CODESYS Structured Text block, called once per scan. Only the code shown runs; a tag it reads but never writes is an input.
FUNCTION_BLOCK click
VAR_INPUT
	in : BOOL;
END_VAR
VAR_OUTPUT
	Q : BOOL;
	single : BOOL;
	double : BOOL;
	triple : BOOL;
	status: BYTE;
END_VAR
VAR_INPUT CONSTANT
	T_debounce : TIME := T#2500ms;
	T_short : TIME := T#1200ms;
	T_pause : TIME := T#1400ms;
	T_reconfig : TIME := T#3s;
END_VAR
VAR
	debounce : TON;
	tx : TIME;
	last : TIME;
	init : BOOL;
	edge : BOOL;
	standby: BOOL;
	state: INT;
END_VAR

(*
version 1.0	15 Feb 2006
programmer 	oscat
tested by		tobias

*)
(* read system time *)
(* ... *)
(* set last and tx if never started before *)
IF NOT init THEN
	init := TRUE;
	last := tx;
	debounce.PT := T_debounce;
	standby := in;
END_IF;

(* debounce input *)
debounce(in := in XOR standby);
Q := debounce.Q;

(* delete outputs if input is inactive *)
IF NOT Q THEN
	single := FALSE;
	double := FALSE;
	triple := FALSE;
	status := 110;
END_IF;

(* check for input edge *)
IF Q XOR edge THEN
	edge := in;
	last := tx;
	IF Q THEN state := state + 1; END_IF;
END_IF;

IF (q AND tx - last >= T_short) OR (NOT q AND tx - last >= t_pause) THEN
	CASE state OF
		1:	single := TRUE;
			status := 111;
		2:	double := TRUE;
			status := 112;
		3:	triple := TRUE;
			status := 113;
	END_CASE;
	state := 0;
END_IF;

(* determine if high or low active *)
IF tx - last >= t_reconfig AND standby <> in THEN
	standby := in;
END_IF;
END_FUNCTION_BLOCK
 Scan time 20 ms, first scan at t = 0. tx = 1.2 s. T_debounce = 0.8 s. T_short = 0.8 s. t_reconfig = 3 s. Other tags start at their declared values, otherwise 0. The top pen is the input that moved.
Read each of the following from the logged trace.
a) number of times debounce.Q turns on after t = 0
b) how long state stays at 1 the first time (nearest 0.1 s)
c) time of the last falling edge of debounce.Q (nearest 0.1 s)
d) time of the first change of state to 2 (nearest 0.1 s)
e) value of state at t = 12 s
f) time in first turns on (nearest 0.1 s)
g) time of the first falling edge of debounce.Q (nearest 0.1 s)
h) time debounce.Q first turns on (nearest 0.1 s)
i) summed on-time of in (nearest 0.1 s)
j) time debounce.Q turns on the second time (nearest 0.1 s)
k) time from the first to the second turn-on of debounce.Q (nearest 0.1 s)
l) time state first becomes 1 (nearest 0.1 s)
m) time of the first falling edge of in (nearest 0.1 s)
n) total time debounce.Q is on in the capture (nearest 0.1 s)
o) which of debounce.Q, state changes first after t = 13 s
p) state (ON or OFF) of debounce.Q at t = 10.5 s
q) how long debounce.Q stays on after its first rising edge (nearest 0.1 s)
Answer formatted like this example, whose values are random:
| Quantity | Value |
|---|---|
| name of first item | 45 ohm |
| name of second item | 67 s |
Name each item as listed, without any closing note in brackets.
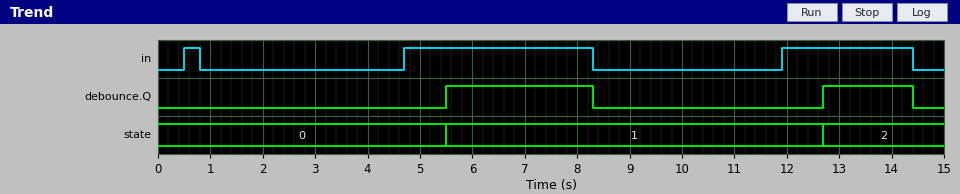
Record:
| Quantity | Value |
|---|---|
| number of times debounce.Q turns on after t = 0 | 2 |
| how long state stays at 1 the first time | 7.2 s |
| time of the last falling edge of debounce.Q | 14.4 s |
| time of the first change of state to 2 | 12.7 s |
| value of state at t = 12 s | 1 |
| time in first turns on | 0.5 s |
| time of the first falling edge of debounce.Q | 8.3 s |
| time debounce.Q first turns on | 5.5 s |
| summed on-time of in | 6.4 s |
| time debounce.Q turns on the second time | 12.7 s |
| time from the first to the second turn-on of debounce.Q | 7.2 s |
| time state first becomes 1 | 5.5 s |
| time of the first falling edge of in | 0.8 s |
| total time debounce.Q is on in the capture | 4.5 s |
| which of debounce.Q, state changes first after t = 13 s | debounce.Q |
| state (ON or OFF) of debounce.Q at t = 10.5 s | OFF |
| how long debounce.Q stays on after its first rising edge | 2.8 s |
